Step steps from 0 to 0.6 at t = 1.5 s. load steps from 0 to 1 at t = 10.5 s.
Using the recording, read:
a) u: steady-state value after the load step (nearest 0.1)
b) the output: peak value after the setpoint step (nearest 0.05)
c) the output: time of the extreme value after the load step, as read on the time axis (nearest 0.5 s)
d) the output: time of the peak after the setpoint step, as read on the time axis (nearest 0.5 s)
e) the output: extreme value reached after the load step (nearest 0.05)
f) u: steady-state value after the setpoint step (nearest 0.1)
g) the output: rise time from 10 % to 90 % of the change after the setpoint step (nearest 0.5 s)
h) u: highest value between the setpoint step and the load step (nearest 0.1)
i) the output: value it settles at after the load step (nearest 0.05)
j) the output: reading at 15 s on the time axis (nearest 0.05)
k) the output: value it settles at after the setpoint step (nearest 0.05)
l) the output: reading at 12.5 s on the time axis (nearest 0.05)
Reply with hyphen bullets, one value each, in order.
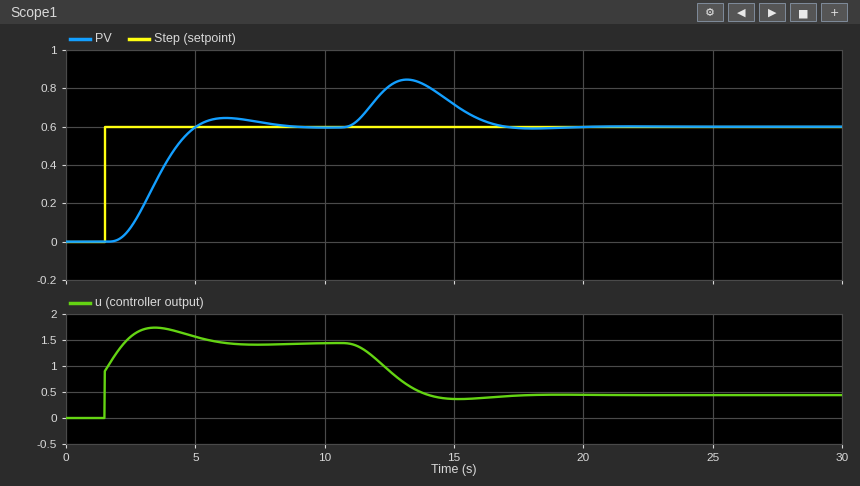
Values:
- 0.4
- 0.65
- 13.0 s
- 6.0 s
- 0.85
- 1.4
- 2.0 s
- 1.7
- 0.60
- 0.70
- 0.60
- 0.80
